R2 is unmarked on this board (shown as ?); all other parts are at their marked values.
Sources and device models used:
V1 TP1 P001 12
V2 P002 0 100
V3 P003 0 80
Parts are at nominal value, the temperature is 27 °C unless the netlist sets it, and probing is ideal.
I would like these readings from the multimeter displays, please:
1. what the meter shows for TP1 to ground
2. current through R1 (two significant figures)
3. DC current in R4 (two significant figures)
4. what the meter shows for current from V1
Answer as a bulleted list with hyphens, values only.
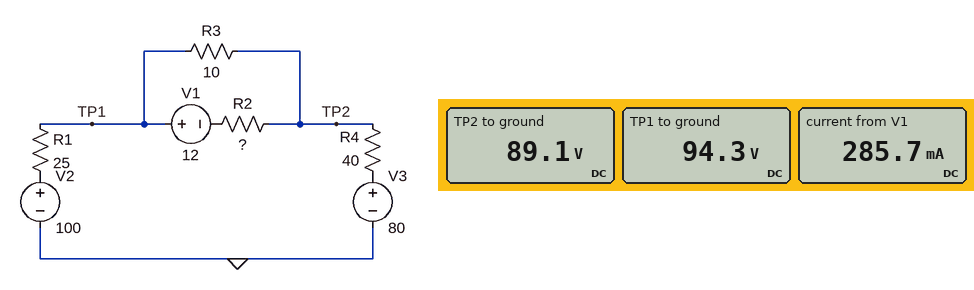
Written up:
- 94.3 V
- 230 mA
- 230 mA
- 285.7 mA
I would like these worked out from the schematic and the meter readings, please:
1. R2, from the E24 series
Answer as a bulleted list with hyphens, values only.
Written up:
- 24 Ω
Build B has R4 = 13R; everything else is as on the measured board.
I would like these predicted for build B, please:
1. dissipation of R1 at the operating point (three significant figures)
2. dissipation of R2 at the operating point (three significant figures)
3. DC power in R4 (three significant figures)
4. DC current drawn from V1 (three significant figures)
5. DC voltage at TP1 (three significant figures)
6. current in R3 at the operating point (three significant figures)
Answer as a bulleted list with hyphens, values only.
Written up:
- 3.34 W
- 1.45 W
- 1.74 W
- 245 mA
- 90.9 V
- 611 mA
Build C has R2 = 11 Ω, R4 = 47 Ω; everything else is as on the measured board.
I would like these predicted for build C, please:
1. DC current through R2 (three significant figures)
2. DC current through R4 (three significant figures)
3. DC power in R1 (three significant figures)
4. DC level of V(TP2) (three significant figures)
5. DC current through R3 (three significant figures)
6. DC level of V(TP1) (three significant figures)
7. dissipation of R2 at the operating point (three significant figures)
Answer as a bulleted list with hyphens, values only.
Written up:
- 483 mA
- 185 mA
- 855 mW
- 88.7 V
- 668 mA
- 95.4 V
- 2.57 W
